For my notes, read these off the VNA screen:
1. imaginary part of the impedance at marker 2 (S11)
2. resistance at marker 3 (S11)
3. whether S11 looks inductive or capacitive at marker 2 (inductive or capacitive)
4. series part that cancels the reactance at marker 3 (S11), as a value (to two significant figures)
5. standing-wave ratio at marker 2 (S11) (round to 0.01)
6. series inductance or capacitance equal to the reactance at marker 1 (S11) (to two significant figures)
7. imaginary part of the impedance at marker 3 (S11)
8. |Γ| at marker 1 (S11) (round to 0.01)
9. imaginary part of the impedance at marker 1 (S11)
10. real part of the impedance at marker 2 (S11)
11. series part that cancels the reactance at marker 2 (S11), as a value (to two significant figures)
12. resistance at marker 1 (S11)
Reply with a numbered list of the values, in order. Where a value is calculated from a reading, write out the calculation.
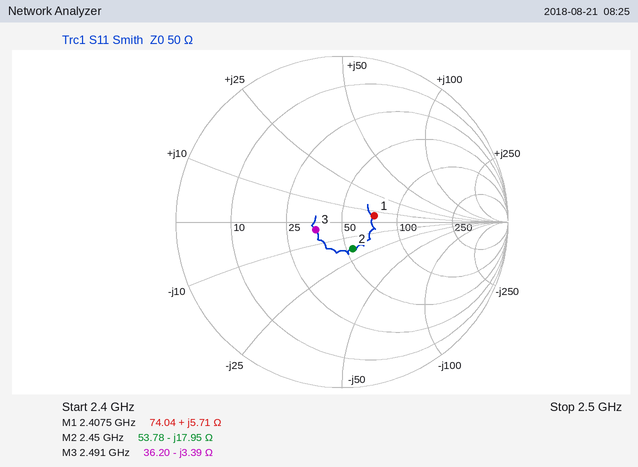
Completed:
1. -17.95 Ω
2. 36.20 Ω
3. capacitive
4. L = 3.39 Ω/(2π × 2.491 GHz) ≈ 217 pH, so 220 pH to two significant figures
5. 1.42
6. L = 5.71 Ω/(2π × 2.4075 GHz) ≈ 377 pH, so 380 pH to two significant figures
7. -3.39 Ω
8. 0.20
9. +5.71 Ω
10. 53.78 Ω
11. L = 17.95 Ω/(2π × 2.45 GHz) ≈ 1.2 nH
12. 74.04 Ω
